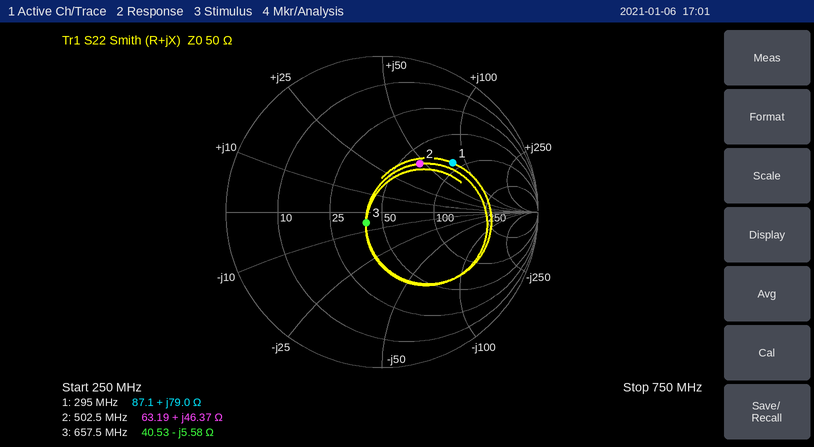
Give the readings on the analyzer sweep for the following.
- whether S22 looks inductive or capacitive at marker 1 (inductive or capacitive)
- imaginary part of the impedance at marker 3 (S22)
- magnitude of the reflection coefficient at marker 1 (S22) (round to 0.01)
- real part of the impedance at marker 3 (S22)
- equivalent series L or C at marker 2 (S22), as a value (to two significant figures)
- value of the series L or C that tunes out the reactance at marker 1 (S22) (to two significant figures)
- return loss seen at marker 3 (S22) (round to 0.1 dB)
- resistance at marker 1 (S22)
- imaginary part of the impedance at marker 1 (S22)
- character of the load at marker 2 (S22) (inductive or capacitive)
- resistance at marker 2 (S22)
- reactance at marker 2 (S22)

inductive
-5.58 Ω
0.55
40.53 Ω
15 nH
6.8 pF
18.3 dB
87.1 Ω
+79.0 Ω
inductive
63.19 Ω
+46.37 Ω
